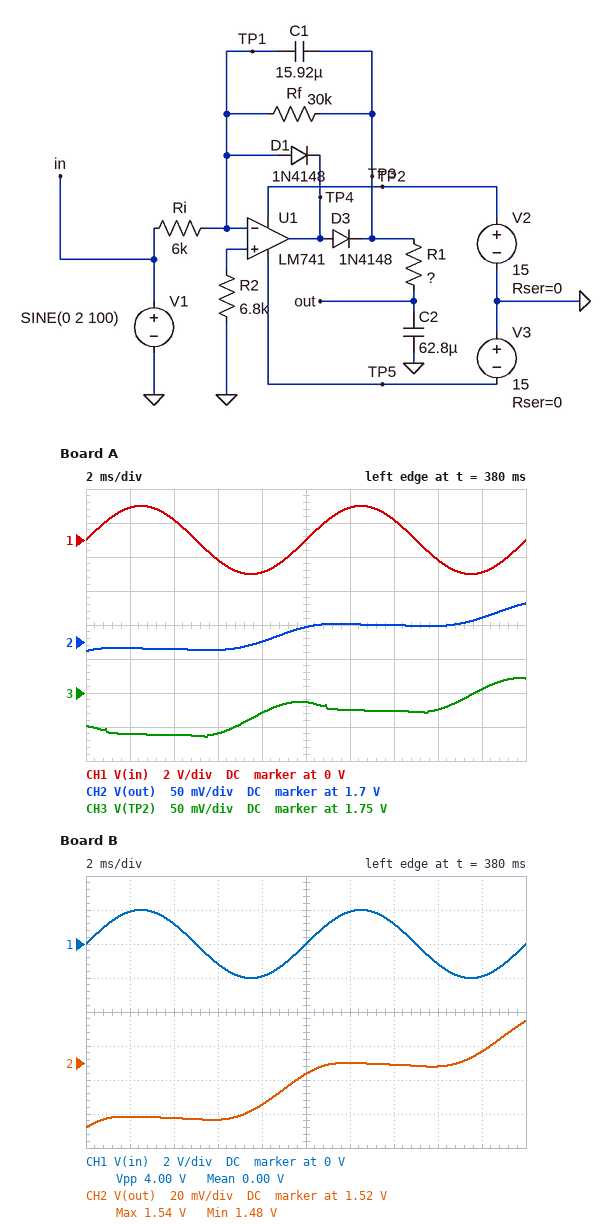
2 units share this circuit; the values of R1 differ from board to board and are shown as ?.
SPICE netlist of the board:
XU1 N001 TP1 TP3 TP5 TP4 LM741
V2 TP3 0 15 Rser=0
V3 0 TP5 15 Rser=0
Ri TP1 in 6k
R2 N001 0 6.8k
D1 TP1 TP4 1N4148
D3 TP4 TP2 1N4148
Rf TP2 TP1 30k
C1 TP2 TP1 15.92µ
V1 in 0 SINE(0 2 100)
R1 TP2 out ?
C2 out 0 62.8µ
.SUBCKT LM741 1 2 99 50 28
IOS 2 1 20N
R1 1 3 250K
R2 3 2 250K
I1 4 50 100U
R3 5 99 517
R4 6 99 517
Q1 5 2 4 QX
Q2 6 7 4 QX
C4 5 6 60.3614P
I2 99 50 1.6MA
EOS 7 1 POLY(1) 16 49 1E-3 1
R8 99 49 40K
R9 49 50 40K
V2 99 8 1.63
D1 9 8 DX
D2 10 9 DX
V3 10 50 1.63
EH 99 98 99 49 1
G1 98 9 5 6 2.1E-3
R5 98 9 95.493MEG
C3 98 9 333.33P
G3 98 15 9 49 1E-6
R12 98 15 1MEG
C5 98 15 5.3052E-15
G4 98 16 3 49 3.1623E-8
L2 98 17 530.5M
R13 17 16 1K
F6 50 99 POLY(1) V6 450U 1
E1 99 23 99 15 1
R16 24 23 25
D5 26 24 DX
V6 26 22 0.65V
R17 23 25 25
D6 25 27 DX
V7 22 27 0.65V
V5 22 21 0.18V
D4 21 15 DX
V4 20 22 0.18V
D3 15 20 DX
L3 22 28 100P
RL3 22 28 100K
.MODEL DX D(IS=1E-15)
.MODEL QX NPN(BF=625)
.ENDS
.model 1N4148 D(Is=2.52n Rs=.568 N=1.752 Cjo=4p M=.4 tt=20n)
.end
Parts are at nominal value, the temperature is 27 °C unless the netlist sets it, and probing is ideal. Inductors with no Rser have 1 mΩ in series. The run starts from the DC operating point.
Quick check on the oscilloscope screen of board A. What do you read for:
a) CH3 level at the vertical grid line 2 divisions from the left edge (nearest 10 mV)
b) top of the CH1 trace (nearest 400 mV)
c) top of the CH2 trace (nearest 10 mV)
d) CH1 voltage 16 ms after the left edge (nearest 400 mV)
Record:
1.69 V
2.0 V
1.76 V
-1.2 V
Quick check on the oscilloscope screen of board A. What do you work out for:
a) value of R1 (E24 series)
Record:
30 Ω
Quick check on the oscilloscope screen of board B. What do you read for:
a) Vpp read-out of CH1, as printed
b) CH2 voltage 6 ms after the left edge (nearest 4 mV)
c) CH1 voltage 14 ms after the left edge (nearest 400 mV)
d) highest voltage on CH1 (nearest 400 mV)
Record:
4.00 V
1.488 V
1.2 V
2.0 V
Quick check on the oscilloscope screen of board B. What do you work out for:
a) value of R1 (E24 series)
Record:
47 Ω
